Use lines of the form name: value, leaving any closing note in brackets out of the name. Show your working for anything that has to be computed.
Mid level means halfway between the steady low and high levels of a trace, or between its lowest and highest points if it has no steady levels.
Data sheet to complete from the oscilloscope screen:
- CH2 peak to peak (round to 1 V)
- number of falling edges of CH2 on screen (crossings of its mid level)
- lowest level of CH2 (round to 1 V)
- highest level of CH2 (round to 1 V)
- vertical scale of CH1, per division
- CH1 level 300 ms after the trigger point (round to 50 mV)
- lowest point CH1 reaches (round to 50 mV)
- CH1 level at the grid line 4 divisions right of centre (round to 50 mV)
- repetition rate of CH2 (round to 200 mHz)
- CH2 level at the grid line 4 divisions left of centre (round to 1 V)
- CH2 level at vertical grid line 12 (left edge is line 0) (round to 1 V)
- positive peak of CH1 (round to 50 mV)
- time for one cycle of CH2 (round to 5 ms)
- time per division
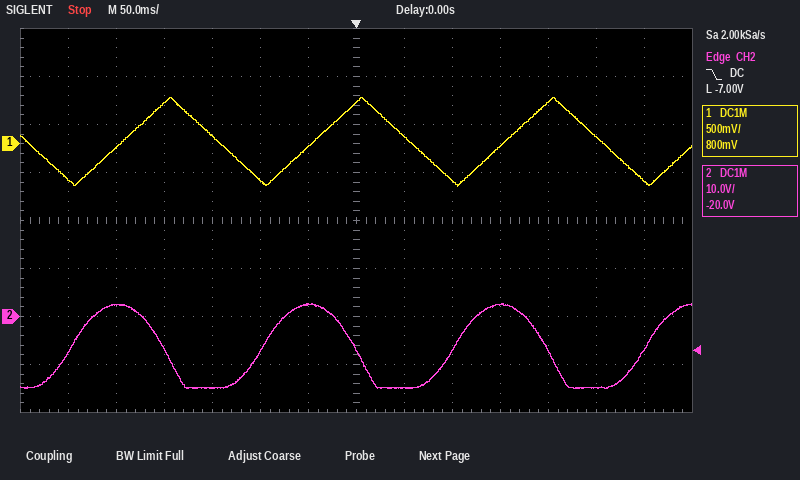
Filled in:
CH2 peak to peak: 3 V − (-15 V) = 18 V
number of falling edges of CH2 on screen: 3
lowest level of CH2: -15 V
highest level of CH2: 3 V
vertical scale of CH1, per division: 500 mV
CH1 level 300 ms after the trigger point: -400 mV
lowest point CH1 reaches: -450 mV
CH1 level at the grid line 4 divisions right of centre: 450 mV
repetition rate of CH2: 1 / 200 ms ≈ 5.0 Hz
CH2 level at the grid line 4 divisions left of centre: -7 V
CH2 level at vertical grid line 12 (left edge is line 0): -15 V
positive peak of CH1: 500 mV
time for one cycle of CH2: 200 ms
time per division: 50 ms
